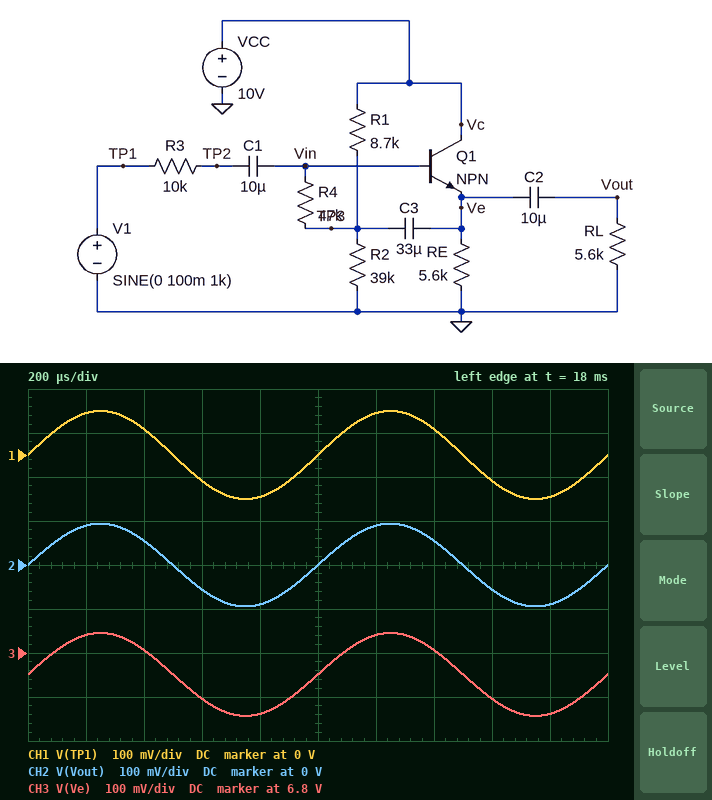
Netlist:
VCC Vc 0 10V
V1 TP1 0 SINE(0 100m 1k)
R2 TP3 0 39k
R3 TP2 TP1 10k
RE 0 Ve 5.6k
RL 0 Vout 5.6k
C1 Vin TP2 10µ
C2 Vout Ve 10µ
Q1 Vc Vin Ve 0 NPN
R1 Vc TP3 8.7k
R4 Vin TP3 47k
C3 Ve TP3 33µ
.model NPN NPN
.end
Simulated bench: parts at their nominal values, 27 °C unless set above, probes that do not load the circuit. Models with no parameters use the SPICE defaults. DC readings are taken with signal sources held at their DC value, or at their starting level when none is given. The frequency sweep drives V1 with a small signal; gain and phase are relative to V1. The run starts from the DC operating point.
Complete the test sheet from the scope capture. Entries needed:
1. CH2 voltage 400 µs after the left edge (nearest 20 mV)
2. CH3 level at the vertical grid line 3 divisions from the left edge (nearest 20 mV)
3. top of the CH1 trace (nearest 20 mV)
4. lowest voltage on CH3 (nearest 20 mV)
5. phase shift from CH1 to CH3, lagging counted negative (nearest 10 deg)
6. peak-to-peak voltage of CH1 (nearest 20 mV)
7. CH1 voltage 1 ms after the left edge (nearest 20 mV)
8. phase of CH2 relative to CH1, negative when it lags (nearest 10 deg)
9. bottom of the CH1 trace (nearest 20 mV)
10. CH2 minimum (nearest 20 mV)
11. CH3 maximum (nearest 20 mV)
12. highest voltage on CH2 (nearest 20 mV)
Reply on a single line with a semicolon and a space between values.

60 mV; 6.70 V; 100 mV; 6.66 V; 0 deg; 200 mV; 0 V; 0 deg; -100 mV; -100 mV; 6.84 V; 100 mV
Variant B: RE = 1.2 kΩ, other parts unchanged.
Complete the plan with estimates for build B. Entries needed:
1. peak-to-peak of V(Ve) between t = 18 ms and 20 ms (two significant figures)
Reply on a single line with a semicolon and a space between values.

180 mV
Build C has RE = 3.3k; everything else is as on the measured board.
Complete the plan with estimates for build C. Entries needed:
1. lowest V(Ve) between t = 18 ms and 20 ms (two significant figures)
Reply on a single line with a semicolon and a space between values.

6.3 V
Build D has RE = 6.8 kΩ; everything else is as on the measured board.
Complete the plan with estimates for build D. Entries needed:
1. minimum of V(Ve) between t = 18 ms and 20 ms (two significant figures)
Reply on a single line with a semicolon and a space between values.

6.8 V
